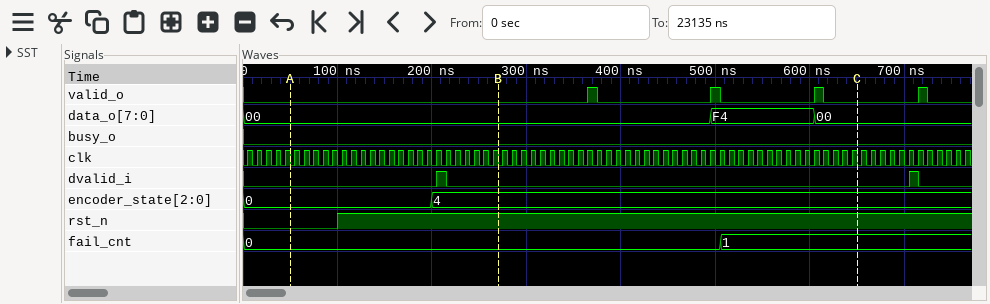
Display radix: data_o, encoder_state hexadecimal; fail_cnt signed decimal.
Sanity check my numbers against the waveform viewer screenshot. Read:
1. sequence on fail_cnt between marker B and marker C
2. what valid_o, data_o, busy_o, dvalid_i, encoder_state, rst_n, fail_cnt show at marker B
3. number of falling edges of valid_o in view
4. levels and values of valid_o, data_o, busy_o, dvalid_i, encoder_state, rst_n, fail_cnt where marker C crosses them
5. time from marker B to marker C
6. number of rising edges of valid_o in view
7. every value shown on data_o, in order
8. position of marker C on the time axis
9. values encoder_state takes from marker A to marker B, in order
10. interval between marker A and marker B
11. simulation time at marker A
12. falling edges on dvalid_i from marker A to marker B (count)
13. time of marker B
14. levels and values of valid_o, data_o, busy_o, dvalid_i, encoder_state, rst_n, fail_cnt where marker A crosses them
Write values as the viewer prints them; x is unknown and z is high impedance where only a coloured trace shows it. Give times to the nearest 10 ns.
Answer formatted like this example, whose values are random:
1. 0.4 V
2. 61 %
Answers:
1. 0, 1
2. valid_o=0, data_o=00, busy_o=0, dvalid_i=0, encoder_state=4, rst_n=1, fail_cnt=0
3. 4
4. valid_o=0, data_o=00, busy_o=0, dvalid_i=0, encoder_state=4, rst_n=1, fail_cnt=1
5. 380 ns
6. 4
7. 00, F4, 00
8. 650 ns
9. 0, 4
10. 220 ns
11. 50 ns
12. 1
13. 270 ns
14. valid_o=0, data_o=00, busy_o=0, dvalid_i=0, encoder_state=0, rst_n=0, fail_cnt=0
